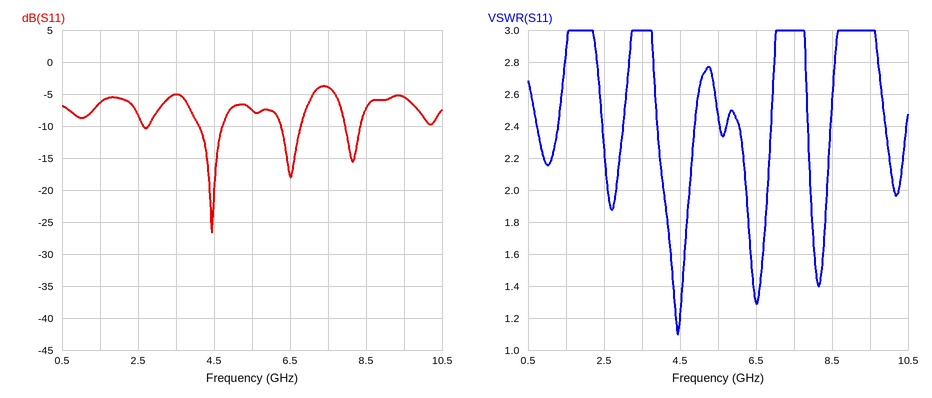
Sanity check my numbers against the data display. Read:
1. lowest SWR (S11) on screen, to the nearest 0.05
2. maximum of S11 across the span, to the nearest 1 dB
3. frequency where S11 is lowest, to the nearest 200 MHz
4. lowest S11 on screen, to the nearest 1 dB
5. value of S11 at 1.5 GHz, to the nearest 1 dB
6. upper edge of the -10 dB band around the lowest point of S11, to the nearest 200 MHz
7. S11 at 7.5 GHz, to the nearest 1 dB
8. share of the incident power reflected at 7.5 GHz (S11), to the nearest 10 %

1.10
-4 dB
4.4 GHz
-27 dB
-6 dB
4.8 GHz
-4 dB
40 %
